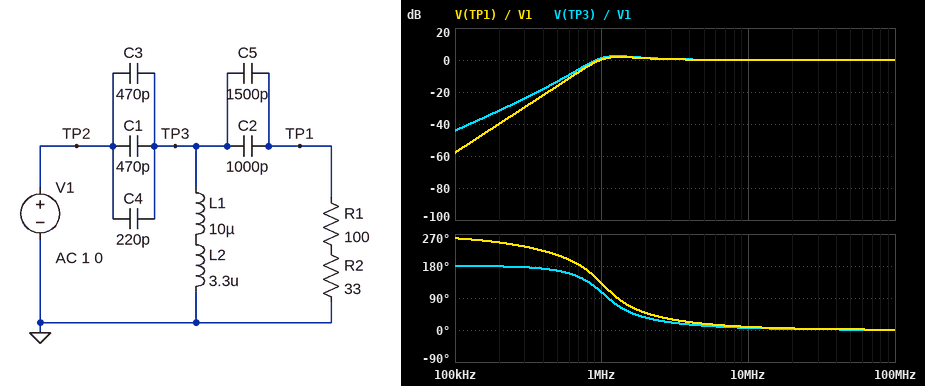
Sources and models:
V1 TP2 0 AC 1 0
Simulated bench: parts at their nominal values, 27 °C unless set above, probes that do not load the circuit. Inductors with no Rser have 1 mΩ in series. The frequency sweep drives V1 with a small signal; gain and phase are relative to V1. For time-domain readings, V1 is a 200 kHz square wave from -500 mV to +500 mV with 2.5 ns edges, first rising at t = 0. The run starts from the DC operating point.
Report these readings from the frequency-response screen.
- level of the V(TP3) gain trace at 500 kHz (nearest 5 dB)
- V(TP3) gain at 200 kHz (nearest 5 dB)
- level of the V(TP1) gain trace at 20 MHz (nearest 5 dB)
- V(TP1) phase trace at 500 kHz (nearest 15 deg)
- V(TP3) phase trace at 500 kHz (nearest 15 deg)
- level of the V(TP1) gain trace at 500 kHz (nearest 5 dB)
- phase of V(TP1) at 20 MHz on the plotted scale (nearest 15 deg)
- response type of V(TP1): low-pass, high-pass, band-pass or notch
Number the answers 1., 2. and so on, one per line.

1. -15 dB
2. -30 dB
3. 0 dB
4. 210 deg
5. 165 deg
6. -15 dB
7. 0 deg
8. high-pass
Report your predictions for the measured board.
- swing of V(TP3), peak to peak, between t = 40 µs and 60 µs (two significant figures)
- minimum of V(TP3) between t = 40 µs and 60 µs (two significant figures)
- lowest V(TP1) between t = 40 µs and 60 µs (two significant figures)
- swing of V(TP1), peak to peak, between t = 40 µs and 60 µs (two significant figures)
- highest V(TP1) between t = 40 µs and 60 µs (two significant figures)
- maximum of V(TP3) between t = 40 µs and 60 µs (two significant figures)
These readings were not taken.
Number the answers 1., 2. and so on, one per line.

1. 2.0 V
2. -990 mV
3. -990 mV
4. 2.0 V
5. 990 mV
6. 990 mV
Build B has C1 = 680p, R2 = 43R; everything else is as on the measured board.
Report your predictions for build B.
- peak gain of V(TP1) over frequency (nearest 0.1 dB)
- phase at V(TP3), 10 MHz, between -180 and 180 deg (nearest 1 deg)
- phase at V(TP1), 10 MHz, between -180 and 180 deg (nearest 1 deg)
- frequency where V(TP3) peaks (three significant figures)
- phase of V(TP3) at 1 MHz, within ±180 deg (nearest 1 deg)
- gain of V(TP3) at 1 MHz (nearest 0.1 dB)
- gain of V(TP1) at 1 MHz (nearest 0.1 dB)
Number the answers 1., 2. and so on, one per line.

1. 3.2 dB
2. 5 deg
3. 7 deg
4. 1.13 MHz
5. 97 deg
6. 3.3 dB
7. 2.5 dB
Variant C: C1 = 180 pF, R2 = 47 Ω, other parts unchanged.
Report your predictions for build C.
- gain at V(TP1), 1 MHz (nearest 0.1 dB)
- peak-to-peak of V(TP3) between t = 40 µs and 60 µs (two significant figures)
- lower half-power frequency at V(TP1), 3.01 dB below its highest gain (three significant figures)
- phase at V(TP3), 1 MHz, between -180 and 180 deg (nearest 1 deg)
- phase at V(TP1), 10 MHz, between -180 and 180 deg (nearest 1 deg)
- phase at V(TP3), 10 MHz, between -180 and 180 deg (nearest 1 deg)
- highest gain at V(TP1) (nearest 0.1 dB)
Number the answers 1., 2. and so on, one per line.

1. -2.9 dB
2. 2.0 V
3. 1.09 MHz
4. 125 deg
5. 10 deg
6. 7 deg
7. 1.6 dB
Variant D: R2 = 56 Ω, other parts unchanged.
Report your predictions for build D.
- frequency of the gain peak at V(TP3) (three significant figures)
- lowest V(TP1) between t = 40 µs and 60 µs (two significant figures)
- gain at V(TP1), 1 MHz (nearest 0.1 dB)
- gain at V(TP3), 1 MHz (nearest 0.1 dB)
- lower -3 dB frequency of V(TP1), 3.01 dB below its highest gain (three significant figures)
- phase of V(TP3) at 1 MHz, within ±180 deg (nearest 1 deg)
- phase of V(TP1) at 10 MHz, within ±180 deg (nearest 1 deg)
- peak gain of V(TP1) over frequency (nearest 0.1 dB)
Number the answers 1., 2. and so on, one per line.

1. 1.28 MHz
2. -990 mV
3. 1.0 dB
4. 1.7 dB
5. 962 kHz
6. 114 deg
7. 7 deg
8. 3.3 dB
